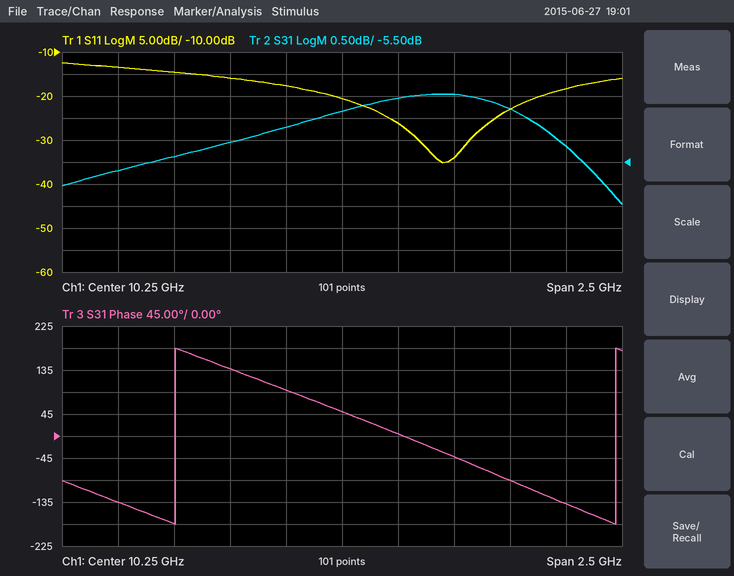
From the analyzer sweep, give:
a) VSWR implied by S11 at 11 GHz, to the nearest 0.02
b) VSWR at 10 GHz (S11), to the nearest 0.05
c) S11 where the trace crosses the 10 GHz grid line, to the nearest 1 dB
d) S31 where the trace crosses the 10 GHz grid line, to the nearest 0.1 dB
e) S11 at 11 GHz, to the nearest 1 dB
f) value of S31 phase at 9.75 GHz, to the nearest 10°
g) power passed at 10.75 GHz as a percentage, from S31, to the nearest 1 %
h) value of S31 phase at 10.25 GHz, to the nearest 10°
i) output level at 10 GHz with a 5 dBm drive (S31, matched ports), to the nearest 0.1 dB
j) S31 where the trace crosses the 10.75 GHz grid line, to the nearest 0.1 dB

1.16
1.30
-18 dB
-4.7 dB
-23 dB
140°
40 %
50°
0.3 dBm
-4.0 dB
